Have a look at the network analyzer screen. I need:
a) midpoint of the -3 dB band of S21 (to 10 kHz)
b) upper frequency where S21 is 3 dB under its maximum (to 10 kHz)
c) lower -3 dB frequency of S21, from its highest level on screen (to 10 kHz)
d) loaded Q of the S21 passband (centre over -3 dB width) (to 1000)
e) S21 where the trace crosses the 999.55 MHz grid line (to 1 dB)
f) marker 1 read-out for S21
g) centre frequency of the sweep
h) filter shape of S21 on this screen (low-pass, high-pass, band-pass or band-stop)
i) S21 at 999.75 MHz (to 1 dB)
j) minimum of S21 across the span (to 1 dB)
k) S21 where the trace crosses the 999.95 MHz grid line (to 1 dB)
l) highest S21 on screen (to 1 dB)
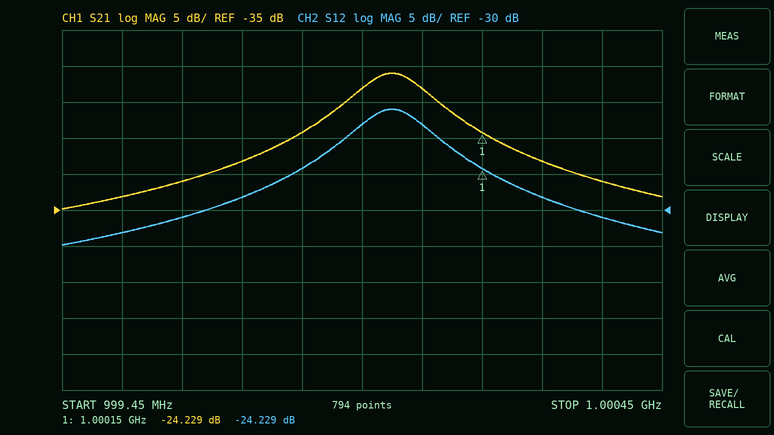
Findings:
1.00000 GHz
1.00006 GHz
999.94 MHz
8000
-33 dB
-24.229 dB
999.95 MHz
band-pass
-28 dB
-35 dB
-18 dB
-16 dB
